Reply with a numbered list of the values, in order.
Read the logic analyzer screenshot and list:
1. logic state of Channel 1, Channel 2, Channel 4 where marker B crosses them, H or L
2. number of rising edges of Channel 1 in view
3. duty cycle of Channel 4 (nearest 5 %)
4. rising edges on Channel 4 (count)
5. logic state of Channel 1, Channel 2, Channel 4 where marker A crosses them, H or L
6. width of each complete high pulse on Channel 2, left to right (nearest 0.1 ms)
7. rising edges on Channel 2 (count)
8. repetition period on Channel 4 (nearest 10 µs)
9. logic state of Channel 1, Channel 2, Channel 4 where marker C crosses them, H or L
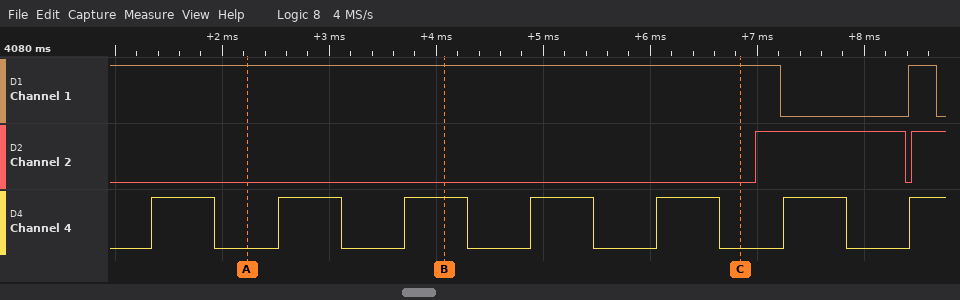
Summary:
1. Channel 1=H, Channel 2=L, Channel 4=H
2. 1
3. 50 %
4. 7
5. Channel 1=H, Channel 2=L, Channel 4=L
6. 1.4 ms
7. 2
8. 1180 µs
9. Channel 1=H, Channel 2=L, Channel 4=L
